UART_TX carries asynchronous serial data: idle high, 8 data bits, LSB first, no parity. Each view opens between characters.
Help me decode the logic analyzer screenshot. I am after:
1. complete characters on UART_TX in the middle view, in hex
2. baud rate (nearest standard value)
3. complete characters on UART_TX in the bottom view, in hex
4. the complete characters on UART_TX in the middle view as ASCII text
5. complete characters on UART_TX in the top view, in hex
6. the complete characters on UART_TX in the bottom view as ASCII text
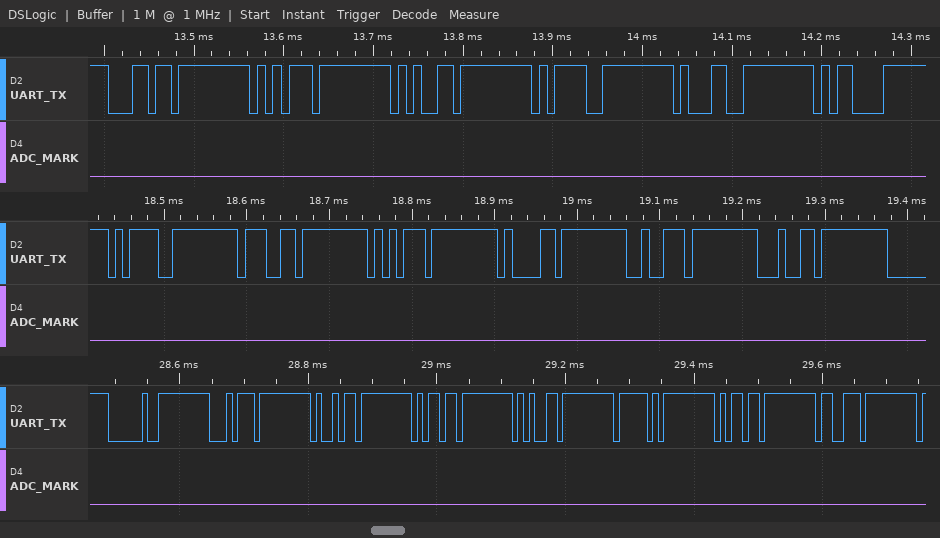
3D, 67, 75, 61, 72, 64
115200 baud
20, 74, 69, 6D, 65, 5F, 6D, 73
"=guard"
6C, 75, 65, 3D, 31, 0D
" time_ms"
